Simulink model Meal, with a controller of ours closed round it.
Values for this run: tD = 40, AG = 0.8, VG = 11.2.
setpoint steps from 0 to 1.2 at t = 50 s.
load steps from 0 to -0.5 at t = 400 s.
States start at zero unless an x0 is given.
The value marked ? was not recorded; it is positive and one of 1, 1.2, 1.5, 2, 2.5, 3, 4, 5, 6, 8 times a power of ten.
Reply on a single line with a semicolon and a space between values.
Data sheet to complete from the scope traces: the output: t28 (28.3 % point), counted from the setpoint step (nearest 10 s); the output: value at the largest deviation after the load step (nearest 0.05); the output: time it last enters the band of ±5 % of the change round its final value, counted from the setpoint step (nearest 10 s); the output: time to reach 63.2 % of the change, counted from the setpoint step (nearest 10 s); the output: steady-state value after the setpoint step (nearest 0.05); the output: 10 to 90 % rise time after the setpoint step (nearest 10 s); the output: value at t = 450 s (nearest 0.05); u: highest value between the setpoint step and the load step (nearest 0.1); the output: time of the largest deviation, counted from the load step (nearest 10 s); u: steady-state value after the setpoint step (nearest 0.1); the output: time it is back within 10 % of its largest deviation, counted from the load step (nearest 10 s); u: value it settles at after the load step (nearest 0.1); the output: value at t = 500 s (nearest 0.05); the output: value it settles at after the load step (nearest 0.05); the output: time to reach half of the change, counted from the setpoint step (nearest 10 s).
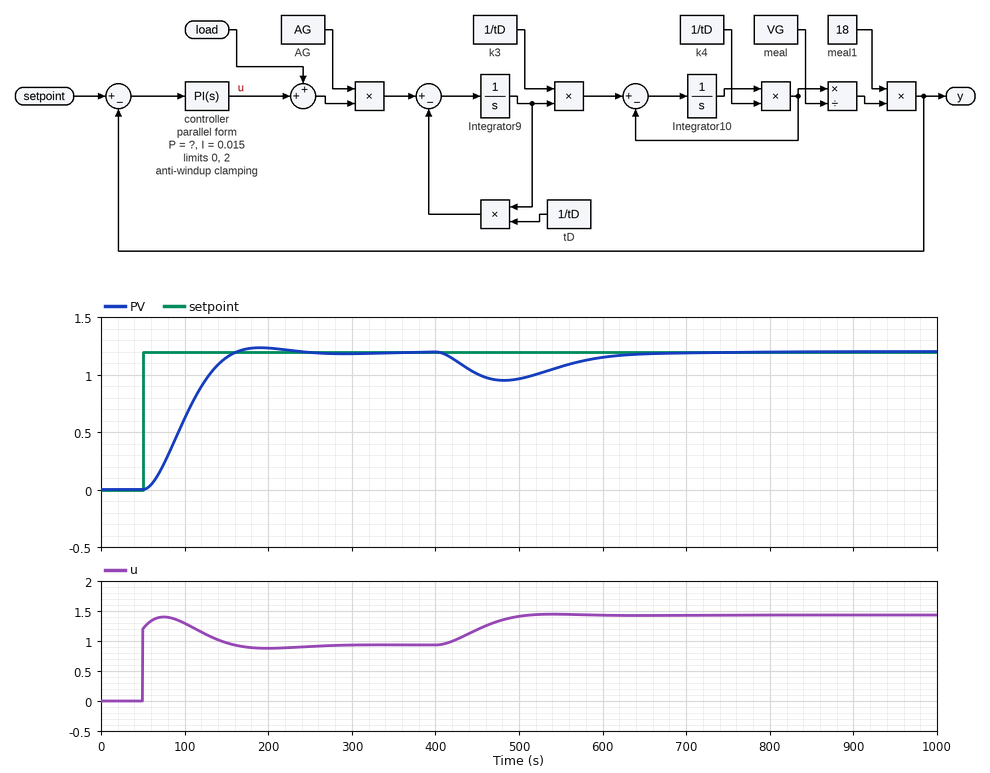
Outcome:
30 s; 0.95; 100 s; 60 s; 1.20; 70 s; 1.00; 1.4; 80 s; 0.9; 240 s; 1.4; 0.95; 1.20; 50 s
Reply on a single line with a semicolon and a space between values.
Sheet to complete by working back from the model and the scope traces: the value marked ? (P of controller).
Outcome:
1
